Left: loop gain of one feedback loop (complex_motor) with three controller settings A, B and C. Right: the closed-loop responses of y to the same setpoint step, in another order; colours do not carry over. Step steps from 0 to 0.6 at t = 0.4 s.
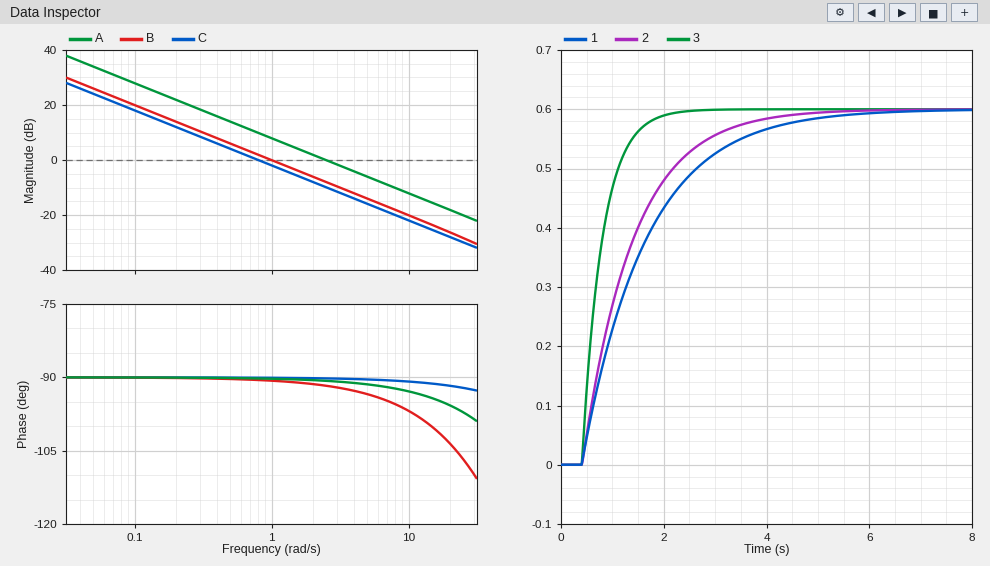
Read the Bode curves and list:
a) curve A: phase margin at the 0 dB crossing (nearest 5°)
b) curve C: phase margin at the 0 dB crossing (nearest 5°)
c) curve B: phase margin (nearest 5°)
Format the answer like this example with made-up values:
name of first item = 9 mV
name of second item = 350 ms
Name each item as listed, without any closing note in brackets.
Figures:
curve A: phase margin at the 0 dB crossing = 90°
curve C: phase margin at the 0 dB crossing = 90°
curve B: phase margin = 90°
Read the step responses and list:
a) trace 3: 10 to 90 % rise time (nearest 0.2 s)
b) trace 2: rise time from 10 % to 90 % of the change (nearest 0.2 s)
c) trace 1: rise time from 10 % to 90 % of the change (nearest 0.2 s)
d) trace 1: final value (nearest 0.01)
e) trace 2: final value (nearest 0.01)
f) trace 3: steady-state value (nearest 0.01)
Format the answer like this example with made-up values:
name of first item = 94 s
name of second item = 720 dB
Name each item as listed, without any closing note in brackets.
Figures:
trace 3: 10 to 90 % rise time = 0.8 s
trace 2: rise time from 10 % to 90 % of the change = 2.2 s
trace 1: rise time from 10 % to 90 % of the change = 2.8 s
trace 1: final value = 0.60
trace 2: final value = 0.60
trace 3: steady-state value = 0.60
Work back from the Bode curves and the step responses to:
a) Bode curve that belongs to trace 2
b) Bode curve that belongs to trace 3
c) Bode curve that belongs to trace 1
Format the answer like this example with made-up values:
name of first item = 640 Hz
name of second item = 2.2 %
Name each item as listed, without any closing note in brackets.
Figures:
Bode curve that belongs to trace 2 = B
Bode curve that belongs to trace 3 = A
Bode curve that belongs to trace 1 = C
